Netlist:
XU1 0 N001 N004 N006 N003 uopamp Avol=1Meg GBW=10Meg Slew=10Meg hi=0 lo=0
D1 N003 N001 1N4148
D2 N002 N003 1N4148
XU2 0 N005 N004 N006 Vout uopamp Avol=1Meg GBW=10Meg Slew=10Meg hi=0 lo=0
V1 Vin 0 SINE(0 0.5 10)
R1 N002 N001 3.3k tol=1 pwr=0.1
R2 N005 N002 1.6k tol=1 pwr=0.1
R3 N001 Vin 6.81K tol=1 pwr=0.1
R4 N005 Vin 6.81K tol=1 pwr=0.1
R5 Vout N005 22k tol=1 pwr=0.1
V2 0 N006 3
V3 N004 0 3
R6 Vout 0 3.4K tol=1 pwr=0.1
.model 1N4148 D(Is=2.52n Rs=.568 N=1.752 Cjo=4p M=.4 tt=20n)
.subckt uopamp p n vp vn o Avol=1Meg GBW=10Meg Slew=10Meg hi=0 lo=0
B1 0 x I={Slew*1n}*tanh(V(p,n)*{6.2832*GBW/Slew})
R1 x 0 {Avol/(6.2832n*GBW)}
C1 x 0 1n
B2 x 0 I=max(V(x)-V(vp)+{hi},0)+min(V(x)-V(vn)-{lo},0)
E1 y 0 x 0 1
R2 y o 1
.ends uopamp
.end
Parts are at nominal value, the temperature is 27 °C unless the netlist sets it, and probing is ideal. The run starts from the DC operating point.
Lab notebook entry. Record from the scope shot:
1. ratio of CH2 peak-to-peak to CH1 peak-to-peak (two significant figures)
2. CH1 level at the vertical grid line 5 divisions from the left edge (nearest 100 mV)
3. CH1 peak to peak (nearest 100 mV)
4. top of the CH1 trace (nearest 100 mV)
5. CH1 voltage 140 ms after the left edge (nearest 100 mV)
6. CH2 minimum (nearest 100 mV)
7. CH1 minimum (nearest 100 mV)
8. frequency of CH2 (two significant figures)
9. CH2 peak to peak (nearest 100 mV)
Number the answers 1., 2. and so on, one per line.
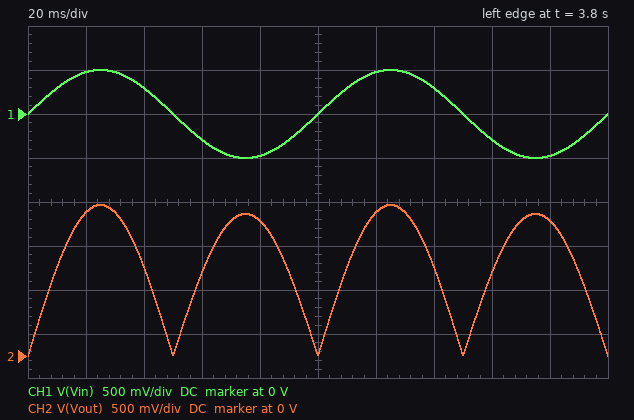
1. 1.7
2. 0 V
3. 1.0 V
4. 500 mV
5. 300 mV
6. 0 V
7. -500 mV
8. 20 Hz
9. 1.7 V
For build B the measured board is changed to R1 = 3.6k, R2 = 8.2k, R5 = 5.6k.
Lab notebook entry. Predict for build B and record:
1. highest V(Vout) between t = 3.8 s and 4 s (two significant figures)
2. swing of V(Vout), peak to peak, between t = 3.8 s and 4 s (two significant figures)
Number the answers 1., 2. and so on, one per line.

1. 410 mV
2. 640 mV
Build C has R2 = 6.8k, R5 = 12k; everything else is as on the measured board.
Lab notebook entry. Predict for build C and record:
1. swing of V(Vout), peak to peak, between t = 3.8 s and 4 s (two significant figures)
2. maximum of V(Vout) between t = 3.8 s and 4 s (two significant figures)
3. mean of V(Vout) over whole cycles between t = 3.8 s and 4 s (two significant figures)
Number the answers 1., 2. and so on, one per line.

1. 1.3 V
2. 880 mV
3. 140 mV
